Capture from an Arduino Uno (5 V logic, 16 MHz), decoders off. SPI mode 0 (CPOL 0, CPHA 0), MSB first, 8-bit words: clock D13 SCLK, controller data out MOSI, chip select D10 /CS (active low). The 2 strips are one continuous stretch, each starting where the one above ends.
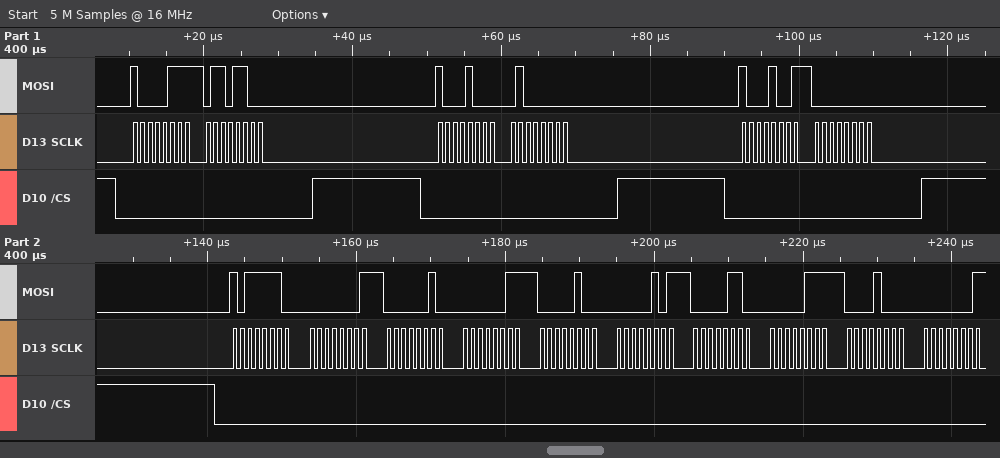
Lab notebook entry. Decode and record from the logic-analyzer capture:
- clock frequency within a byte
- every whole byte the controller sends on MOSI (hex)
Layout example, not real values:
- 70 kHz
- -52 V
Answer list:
- 1 MHz
- 87 6C 88 40 89 00 BE 01 02 03 04 05 06 07 08 01
